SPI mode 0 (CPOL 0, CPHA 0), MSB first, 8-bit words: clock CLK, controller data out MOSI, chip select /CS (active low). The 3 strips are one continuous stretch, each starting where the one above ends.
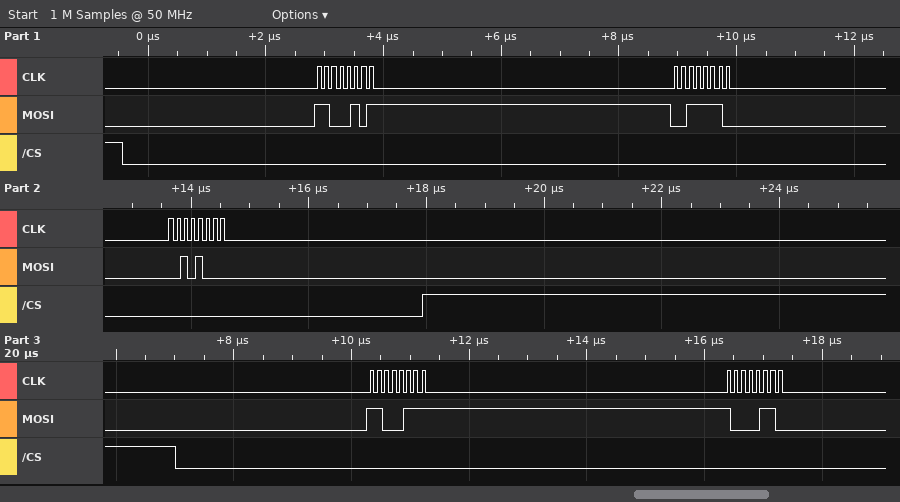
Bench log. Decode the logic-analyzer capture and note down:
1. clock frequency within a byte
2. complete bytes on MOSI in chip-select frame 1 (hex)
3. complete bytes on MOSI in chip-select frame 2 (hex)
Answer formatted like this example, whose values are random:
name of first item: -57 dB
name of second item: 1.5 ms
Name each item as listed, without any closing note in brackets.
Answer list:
clock frequency within a byte: 8 MHz
complete bytes on MOSI in chip-select frame 1: C5 3E 28
complete bytes on MOSI in chip-select frame 2: C7 86
